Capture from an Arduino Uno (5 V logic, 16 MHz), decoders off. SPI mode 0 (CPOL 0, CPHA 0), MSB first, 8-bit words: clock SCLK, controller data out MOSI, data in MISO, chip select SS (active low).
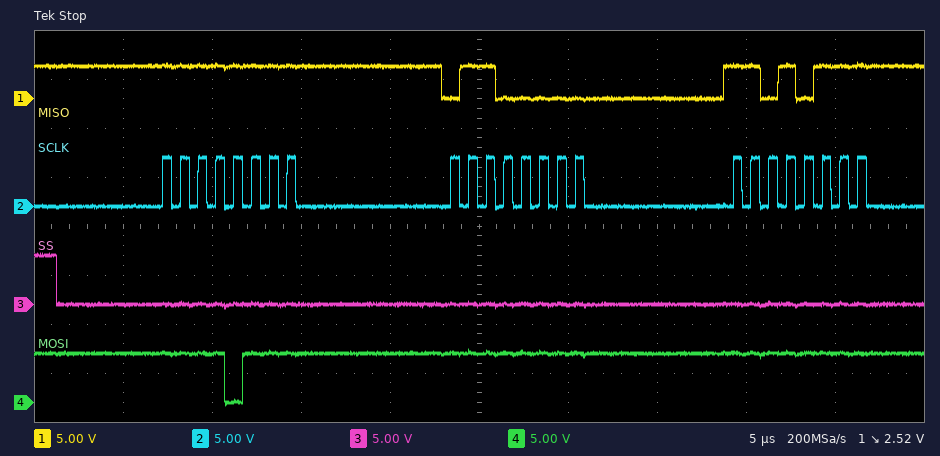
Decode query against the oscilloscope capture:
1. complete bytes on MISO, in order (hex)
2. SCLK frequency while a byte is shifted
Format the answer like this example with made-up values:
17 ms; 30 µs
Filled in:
0xFF 0x60 0xD7; 1 MHz
